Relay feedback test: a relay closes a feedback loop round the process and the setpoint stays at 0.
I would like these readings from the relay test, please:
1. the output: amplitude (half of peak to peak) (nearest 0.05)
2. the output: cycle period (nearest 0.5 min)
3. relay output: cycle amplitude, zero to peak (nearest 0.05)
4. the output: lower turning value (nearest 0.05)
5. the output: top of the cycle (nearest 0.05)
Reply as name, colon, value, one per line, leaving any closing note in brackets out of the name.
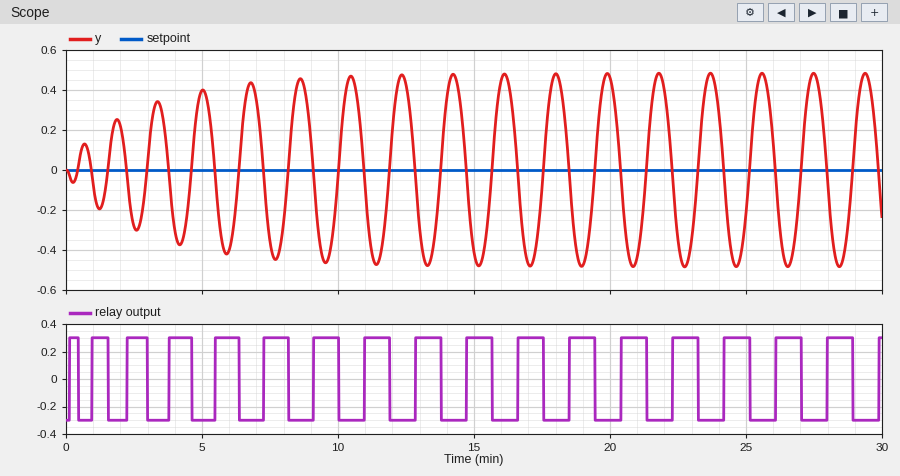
the output: amplitude (half of peak to peak): 0.50
the output: cycle period: 2.0 min
relay output: cycle amplitude, zero to peak: 0.30
the output: lower turning value: -0.50
the output: top of the cycle: 0.50
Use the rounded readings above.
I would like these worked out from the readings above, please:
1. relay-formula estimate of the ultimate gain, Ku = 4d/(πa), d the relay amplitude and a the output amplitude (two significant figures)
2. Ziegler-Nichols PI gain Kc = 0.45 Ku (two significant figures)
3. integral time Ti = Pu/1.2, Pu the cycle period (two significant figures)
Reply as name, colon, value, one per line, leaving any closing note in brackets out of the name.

relay-formula estimate of the ultimate gain, Ku = 4d/(πa), d the relay amplitude and a the output amplitude: 0.76
Ziegler-Nichols PI gain Kc = 0.45 Ku: 0.34
integral time Ti = Pu/1.2, Pu the cycle period: 1.7 min
